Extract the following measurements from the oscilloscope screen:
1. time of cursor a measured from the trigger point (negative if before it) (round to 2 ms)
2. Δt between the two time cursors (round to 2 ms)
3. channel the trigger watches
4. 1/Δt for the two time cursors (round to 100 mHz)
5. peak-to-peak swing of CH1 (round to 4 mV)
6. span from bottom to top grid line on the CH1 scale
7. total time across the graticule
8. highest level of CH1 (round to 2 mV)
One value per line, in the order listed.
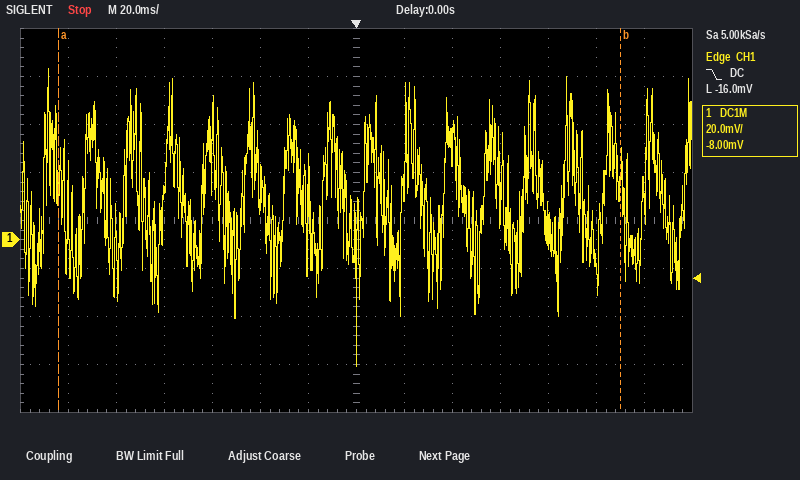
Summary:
-124 ms
234 ms
CH1
4.3 Hz
124 mV
160 mV
280 ms
72 mV
